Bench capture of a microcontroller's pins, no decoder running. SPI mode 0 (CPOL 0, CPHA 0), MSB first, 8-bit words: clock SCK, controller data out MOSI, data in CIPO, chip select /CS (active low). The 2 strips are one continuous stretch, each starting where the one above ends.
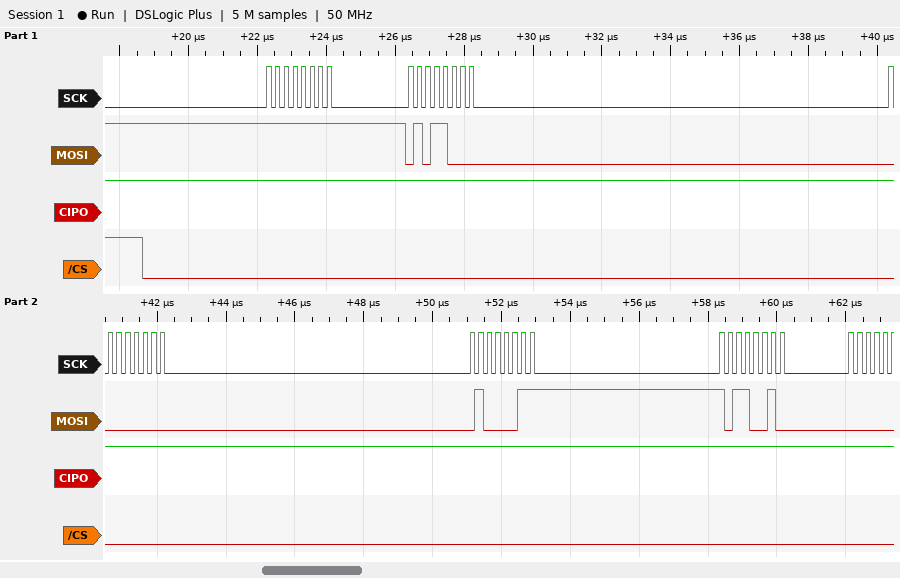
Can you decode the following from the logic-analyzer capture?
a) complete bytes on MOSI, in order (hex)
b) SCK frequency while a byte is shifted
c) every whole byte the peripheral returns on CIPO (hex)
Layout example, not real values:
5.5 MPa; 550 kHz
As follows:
0xFF 0x58 0x00 0x43 0xB2; 4 MHz; 0xFF 0xFF 0xFF 0xFF 0xFF
